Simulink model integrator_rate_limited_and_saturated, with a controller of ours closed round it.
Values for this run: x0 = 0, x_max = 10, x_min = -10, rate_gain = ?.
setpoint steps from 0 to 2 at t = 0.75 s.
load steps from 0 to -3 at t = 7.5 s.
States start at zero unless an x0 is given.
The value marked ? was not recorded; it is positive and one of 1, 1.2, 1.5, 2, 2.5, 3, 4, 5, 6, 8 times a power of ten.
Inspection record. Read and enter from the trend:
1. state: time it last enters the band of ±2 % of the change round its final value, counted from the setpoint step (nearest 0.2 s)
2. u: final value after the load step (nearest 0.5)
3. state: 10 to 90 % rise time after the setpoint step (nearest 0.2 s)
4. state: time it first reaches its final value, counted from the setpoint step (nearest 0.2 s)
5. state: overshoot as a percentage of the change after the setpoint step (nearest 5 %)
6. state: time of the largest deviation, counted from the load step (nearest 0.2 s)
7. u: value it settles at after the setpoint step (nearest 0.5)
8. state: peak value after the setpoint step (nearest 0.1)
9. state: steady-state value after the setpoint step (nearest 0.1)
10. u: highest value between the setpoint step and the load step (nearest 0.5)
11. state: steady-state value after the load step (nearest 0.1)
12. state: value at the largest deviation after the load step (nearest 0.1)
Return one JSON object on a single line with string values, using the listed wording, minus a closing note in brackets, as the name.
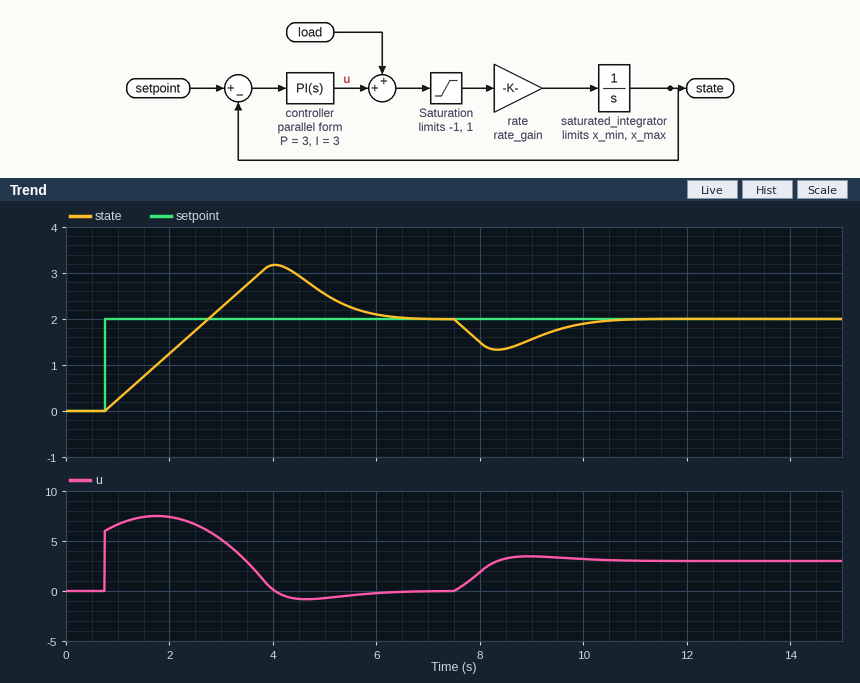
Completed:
{"state: time it last enters the band of ±2 % of the change round its final value, counted from the setpoint step": "5.6 s", "u: final value after the load step": "3.0", "state: 10 to 90 % rise time after the setpoint step": "1.6 s", "state: time it first reaches its final value, counted from the setpoint step": "2.0 s", "state: overshoot as a percentage of the change after the setpoint step": "60 %", "state: time of the largest deviation, counted from the load step": "0.8 s", "u: value it settles at after the setpoint step": "0.0", "state: peak value after the setpoint step": "3.2", "state: steady-state value after the setpoint step": "2.0", "u: highest value between the setpoint step and the load step": "7.5", "state: steady-state value after the load step": "2.0", "state: value at the largest deviation after the load step": "1.3"}
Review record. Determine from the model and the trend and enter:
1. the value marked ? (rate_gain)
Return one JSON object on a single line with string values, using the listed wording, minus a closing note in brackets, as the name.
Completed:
{"the value marked ?": "1"}
